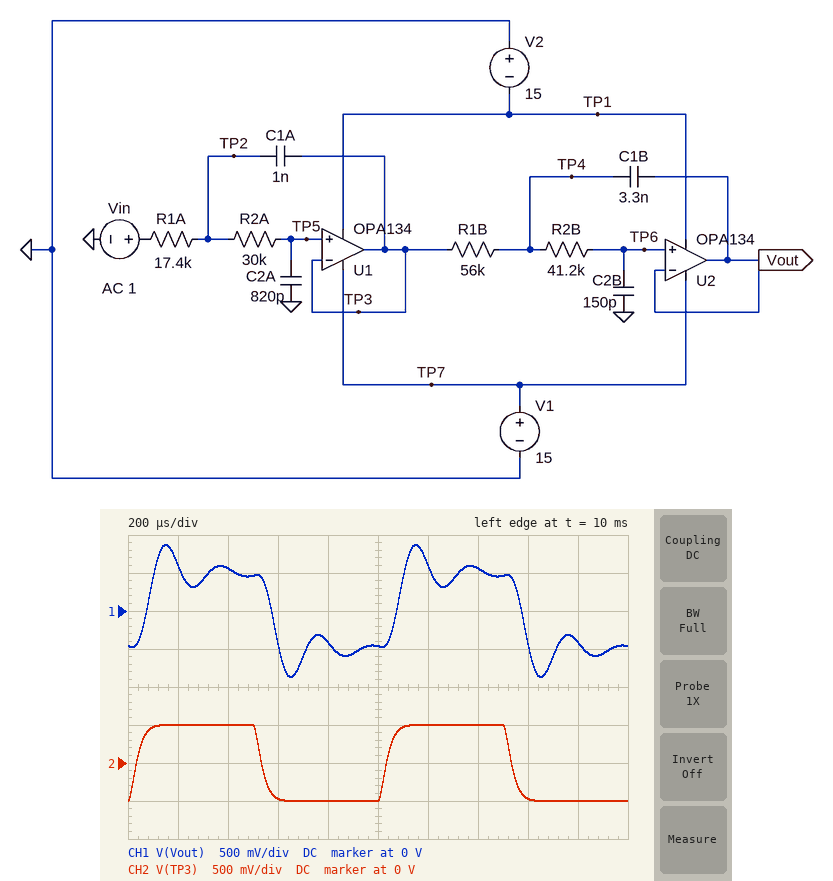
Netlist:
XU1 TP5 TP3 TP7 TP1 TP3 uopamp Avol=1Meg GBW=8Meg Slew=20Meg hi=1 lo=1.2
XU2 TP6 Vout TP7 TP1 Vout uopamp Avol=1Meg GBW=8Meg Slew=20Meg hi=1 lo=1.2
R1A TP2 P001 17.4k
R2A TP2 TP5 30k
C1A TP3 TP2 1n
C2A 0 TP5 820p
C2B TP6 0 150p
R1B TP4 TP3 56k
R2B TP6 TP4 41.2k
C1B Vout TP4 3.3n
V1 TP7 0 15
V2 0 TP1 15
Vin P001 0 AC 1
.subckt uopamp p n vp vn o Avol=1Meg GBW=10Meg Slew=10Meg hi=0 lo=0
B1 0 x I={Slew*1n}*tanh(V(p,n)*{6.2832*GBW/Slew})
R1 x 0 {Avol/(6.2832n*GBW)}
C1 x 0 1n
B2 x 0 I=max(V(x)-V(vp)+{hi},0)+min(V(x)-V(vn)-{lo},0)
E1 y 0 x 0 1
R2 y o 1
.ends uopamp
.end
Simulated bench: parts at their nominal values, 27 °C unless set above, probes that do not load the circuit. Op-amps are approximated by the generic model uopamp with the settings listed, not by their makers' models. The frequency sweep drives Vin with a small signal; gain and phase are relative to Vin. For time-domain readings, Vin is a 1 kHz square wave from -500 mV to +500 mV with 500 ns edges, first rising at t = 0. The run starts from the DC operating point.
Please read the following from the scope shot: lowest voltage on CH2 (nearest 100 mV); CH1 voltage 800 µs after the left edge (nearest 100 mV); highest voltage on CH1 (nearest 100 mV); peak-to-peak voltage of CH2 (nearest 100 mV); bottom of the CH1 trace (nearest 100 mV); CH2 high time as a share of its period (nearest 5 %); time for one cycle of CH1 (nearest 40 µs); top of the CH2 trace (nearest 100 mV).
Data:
-500 mV
-400 mV
900 mV
1.0 V
-900 mV
50 %
1.00 ms
500 mV
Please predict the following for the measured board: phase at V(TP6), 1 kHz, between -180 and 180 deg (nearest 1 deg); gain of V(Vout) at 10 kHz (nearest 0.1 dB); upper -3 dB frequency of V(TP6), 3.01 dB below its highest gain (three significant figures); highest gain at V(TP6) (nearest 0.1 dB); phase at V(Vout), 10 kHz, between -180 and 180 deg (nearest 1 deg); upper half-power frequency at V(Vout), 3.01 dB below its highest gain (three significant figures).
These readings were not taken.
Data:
-19 deg
-19.3 dB
5.26 kHz
5.4 dB
89 deg
5.26 kHz
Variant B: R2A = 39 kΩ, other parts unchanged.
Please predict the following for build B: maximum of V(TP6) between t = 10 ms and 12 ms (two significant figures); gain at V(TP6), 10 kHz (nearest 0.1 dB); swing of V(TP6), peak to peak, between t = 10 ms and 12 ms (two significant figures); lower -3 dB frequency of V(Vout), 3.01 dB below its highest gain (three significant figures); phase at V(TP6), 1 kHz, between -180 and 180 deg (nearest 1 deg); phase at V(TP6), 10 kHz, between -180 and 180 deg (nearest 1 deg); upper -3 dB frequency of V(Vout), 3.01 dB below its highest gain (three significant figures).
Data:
820 mV
-21.2 dB
1.6 V
2.61 kHz
-22 deg
82 deg
5.22 kHz
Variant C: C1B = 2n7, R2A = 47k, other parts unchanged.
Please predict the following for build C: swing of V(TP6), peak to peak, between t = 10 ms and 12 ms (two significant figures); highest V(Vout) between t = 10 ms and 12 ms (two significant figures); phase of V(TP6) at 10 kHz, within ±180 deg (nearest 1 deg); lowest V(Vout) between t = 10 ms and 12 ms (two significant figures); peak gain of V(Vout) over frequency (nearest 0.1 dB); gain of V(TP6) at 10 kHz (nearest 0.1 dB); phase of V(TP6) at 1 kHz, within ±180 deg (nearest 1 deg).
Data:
1.4 V
720 mV
82 deg
-720 mV
2.5 dB
-20.5 dB
-24 deg
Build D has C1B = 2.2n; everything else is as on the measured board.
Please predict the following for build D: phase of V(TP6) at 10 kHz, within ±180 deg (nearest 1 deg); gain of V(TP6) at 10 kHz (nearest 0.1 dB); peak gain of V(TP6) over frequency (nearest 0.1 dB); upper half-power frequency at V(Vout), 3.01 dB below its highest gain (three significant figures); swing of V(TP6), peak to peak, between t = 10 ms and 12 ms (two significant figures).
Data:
99 deg
-15.0 dB
3.1 dB
6.37 kHz
1.5 V
